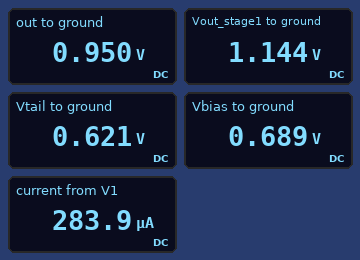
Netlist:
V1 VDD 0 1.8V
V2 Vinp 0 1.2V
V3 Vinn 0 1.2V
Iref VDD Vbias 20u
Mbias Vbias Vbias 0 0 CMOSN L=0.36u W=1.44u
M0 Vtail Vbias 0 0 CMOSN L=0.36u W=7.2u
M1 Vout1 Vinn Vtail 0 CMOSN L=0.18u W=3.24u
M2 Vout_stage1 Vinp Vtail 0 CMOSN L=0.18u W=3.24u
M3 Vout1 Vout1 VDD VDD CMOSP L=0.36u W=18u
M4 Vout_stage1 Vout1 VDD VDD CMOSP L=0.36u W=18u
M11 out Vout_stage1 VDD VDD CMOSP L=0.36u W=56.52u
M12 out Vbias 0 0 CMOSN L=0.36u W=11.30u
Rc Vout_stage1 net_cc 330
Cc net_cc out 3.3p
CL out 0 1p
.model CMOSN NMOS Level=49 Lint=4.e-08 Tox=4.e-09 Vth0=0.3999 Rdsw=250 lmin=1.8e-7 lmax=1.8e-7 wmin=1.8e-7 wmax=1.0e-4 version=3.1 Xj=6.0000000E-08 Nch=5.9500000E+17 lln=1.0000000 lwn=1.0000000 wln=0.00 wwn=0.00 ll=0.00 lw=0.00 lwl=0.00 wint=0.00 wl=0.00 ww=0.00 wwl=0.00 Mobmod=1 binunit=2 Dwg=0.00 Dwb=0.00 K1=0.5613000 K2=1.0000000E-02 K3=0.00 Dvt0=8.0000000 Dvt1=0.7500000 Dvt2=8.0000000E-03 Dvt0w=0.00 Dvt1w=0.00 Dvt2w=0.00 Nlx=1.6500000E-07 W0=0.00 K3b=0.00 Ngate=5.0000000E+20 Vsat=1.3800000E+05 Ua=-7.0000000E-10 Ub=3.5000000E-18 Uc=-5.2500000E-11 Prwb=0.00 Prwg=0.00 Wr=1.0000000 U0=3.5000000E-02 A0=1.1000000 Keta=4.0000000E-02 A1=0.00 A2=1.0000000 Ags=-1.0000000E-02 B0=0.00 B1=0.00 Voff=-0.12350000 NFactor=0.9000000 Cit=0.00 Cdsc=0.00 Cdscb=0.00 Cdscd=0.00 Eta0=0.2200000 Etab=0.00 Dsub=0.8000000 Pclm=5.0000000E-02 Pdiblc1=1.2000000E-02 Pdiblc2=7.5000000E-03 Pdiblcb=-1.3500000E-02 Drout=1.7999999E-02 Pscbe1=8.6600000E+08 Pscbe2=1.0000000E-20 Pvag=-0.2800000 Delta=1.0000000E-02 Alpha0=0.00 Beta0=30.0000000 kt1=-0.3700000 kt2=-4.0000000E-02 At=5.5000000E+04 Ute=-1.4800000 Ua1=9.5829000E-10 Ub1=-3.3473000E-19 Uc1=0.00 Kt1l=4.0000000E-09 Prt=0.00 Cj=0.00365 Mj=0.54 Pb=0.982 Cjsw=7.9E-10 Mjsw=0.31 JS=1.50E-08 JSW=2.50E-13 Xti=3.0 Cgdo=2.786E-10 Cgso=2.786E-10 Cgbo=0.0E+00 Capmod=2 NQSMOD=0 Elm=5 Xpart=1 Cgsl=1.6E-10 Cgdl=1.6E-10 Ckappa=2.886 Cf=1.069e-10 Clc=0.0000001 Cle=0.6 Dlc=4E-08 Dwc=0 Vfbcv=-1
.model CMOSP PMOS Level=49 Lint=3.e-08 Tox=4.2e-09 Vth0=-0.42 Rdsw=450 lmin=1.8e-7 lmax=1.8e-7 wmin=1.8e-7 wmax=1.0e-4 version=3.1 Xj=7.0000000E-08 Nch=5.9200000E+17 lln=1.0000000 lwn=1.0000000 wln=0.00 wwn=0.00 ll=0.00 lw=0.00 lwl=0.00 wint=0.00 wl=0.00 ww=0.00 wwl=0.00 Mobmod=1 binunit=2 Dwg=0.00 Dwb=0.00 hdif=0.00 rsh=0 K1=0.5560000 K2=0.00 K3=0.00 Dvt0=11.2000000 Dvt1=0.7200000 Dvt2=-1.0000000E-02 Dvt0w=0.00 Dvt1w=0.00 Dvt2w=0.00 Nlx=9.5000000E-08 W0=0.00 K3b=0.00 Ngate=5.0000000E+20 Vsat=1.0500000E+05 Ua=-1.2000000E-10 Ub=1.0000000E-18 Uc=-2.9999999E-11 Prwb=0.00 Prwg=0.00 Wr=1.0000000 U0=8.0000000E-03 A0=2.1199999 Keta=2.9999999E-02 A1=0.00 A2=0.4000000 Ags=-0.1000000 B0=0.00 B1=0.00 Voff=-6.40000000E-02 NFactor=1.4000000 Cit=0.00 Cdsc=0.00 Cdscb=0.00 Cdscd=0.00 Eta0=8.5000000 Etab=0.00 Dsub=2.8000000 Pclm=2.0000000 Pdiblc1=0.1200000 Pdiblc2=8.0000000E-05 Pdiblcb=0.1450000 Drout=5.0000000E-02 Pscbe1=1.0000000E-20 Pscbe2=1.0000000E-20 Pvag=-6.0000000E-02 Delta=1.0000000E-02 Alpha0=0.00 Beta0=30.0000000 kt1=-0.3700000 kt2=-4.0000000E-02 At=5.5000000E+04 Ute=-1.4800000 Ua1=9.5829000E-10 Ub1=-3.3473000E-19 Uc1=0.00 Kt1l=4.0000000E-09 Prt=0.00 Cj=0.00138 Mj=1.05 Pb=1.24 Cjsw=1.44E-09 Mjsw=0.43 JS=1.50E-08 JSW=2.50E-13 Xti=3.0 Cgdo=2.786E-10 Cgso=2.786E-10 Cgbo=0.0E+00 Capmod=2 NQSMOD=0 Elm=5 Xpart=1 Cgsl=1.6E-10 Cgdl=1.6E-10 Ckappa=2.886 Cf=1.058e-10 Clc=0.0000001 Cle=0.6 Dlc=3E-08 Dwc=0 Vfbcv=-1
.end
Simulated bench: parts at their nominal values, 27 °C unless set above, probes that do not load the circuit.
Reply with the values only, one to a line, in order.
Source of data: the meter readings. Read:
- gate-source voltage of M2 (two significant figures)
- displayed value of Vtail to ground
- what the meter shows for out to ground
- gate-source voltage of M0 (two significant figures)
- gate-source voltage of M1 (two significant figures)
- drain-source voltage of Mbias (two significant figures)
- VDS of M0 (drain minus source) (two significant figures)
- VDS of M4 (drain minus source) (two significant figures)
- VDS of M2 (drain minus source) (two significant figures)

580 mV
0.621 V
0.950 V
690 mV
580 mV
690 mV
620 mV
-660 mV
520 mV
